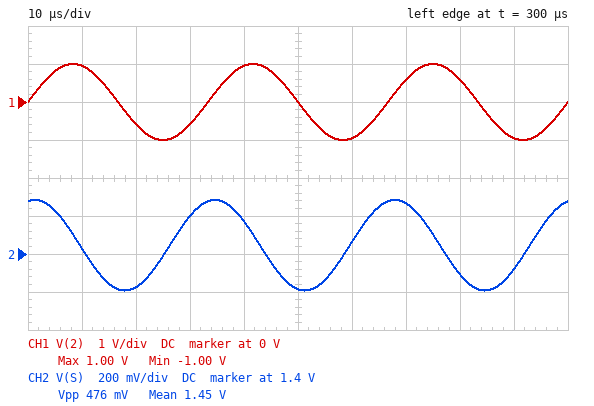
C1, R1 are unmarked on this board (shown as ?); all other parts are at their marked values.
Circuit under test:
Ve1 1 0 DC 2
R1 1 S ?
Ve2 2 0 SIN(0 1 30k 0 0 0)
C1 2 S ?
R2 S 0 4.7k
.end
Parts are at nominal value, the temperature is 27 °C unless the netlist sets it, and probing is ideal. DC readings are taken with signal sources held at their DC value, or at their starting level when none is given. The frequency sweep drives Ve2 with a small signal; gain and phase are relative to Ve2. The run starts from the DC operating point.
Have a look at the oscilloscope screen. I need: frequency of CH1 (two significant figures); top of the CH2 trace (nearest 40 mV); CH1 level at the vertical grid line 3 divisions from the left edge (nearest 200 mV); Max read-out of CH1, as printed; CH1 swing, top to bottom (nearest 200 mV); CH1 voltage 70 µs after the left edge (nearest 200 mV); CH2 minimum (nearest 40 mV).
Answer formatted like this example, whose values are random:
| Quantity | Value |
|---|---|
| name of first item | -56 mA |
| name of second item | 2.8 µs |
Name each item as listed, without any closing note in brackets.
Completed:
| Quantity | Value |
|---|---|
| frequency of CH1 | 30 kHz |
| top of the CH2 trace | 1.68 V |
| CH1 level at the vertical grid line 3 divisions from the left edge | -600 mV |
| Max read-out of CH1, as printed | 1.00 V |
| CH1 swing, top to bottom | 2.0 V |
| CH1 voltage 70 µs after the left edge | 600 mV |
| CH2 minimum | 1.20 V |
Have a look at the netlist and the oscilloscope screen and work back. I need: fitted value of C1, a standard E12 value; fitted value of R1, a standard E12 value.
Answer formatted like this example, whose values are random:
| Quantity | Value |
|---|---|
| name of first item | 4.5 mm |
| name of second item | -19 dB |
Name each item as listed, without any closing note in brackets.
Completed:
| Quantity | Value |
|---|---|
| fitted value of C1, a standard E12 value | 1 nF |
| fitted value of R1, a standard E12 value | 1.8 kΩ |
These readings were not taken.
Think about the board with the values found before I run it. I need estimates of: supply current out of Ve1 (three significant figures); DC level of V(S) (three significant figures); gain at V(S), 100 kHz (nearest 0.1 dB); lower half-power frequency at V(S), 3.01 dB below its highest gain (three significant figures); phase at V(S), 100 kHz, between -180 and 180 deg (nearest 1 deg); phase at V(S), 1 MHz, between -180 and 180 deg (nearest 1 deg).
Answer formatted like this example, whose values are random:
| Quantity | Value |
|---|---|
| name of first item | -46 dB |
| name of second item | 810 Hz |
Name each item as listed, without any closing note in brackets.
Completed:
| Quantity | Value |
|---|---|
| supply current out of Ve1 | 308 µA |
| DC level of V(S) | 1.45 V |
| gain at V(S), 100 kHz | -4.0 dB |
| lower half-power frequency at V(S), 3.01 dB below its highest gain | 122 kHz |
| phase at V(S), 100 kHz, between -180 and 180 deg | 51 deg |
| phase at V(S), 1 MHz, between -180 and 180 deg | 7 deg |
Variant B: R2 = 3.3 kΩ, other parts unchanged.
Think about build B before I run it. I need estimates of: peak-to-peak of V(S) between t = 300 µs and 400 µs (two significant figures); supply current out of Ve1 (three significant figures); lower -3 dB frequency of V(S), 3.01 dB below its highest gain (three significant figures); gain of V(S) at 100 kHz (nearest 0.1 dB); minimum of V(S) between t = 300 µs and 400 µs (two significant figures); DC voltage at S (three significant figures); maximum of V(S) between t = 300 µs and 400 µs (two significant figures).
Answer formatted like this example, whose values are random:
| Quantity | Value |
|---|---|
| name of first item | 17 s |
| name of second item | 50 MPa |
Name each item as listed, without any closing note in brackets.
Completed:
| Quantity | Value |
|---|---|
| peak-to-peak of V(S) between t = 300 µs and 400 µs | 430 mV |
| supply current out of Ve1 | 392 µA |
| lower -3 dB frequency of V(S), 3.01 dB below its highest gain | 137 kHz |
| gain of V(S) at 100 kHz | -4.6 dB |
| minimum of V(S) between t = 300 µs and 400 µs | 1.1 V |
| DC voltage at S | 1.29 V |
| maximum of V(S) between t = 300 µs and 400 µs | 1.5 V |
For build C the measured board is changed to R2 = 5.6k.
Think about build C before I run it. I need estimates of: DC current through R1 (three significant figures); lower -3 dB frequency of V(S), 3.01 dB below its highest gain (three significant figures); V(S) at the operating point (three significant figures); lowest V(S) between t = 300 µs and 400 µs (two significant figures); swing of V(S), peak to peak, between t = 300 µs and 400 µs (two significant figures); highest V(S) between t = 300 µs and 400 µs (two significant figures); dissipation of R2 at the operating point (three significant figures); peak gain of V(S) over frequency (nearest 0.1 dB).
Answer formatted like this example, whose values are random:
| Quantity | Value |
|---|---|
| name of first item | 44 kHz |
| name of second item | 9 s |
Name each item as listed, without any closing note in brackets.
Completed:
| Quantity | Value |
|---|---|
| DC current through R1 | 270 µA |
| lower -3 dB frequency of V(S), 3.01 dB below its highest gain | 117 kHz |
| V(S) at the operating point | 1.51 V |
| lowest V(S) between t = 300 µs and 400 µs | 1.3 V |
| swing of V(S), peak to peak, between t = 300 µs and 400 µs | 500 mV |
| highest V(S) between t = 300 µs and 400 µs | 1.8 V |
| dissipation of R2 at the operating point | 409 µW |
| peak gain of V(S) over frequency | 0 dB |
